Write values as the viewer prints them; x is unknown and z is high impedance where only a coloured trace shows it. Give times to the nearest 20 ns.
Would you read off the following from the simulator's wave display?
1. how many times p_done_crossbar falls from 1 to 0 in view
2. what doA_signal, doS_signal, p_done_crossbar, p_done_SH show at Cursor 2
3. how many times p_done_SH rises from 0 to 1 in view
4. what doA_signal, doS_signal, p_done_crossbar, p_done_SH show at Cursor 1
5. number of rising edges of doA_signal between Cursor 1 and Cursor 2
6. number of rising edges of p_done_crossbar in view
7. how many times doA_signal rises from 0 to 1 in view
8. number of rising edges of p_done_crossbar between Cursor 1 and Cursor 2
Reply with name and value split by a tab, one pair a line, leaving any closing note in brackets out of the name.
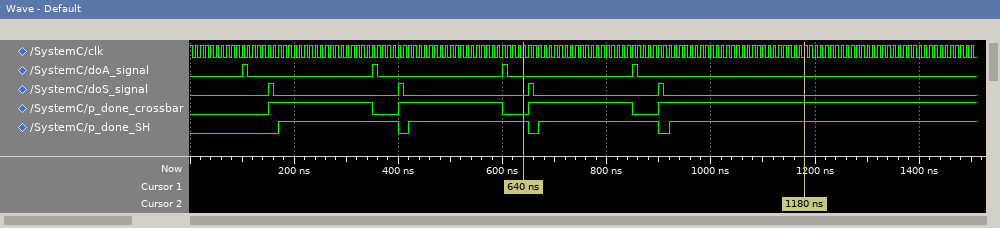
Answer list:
how many times p_done_crossbar falls from 1 to 0 in view	3
what doA_signal, doS_signal, p_done_crossbar, p_done_SH show at Cursor 2	doA_signal=0, doS_signal=0, p_done_crossbar=1, p_done_SH=1
how many times p_done_SH rises from 0 to 1 in view	4
what doA_signal, doS_signal, p_done_crossbar, p_done_SH show at Cursor 1	doA_signal=0, doS_signal=0, p_done_crossbar=0, p_done_SH=1
number of rising edges of doA_signal between Cursor 1 and Cursor 2	1
number of rising edges of p_done_crossbar in view	4
how many times doA_signal rises from 0 to 1 in view	4
number of rising edges of p_done_crossbar between Cursor 1 and Cursor 2	2
